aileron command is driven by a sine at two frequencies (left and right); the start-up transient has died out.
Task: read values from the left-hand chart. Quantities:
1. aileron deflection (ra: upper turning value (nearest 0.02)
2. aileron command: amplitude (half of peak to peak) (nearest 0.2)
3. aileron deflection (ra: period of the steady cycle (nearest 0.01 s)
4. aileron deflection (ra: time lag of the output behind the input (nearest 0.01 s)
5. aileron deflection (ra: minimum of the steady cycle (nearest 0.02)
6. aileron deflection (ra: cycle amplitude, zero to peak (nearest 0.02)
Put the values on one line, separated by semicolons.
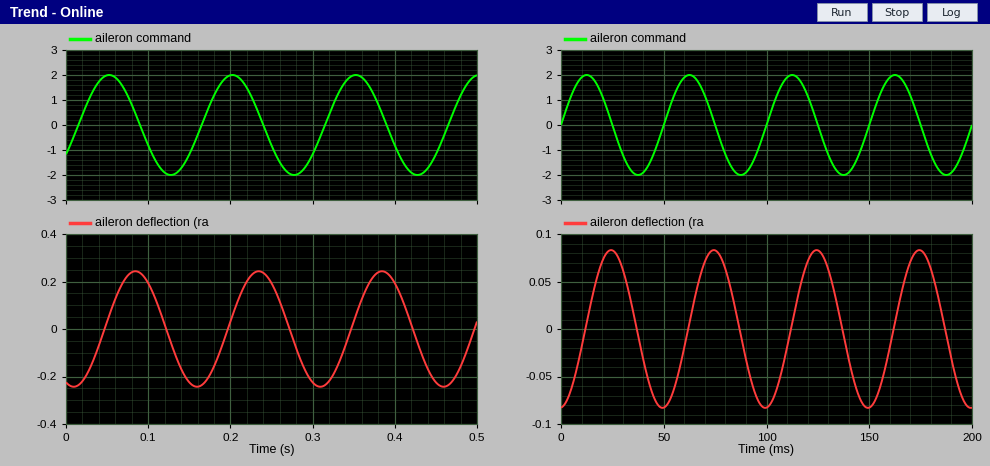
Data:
0.24; 2.0; 0.15 s; 0.03 s; -0.24; 0.24
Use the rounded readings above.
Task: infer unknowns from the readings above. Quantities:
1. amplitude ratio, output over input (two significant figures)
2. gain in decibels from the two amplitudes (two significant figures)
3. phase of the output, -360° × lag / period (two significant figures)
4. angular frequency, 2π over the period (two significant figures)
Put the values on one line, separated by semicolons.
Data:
0.12; -18 dB; -72°; 42 rad/s
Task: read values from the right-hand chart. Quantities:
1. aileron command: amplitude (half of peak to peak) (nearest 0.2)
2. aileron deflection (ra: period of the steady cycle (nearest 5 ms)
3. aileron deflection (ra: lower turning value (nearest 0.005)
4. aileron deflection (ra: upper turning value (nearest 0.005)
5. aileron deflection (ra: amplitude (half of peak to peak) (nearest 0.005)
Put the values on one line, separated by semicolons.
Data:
2.0; 50 ms; -0.085; 0.085; 0.085
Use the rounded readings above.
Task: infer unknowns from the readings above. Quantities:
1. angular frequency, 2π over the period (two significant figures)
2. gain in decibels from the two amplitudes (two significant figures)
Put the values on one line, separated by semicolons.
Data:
0.13 rad/ms; -27 dB
